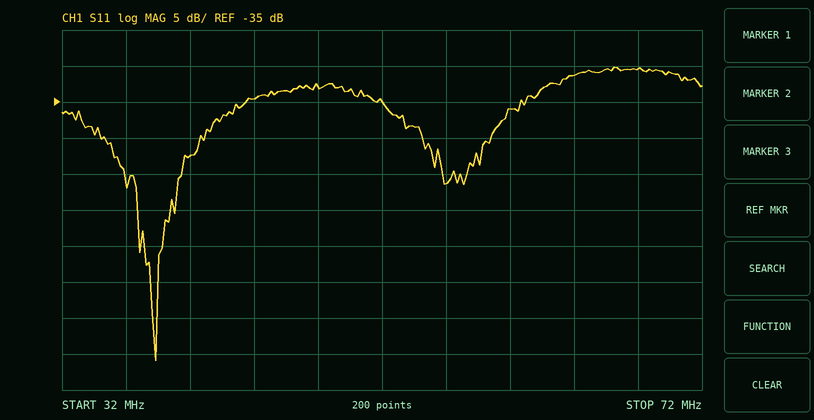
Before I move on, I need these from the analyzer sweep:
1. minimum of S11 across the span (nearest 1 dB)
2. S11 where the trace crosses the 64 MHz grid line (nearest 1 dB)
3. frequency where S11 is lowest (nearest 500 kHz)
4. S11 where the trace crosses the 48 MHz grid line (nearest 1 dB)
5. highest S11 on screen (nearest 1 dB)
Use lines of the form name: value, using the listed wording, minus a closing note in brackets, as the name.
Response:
minimum of S11 across the span: -71 dB
S11 where the trace crosses the 64 MHz grid line: -31 dB
frequency where S11 is lowest: 38.0 MHz
S11 where the trace crosses the 48 MHz grid line: -33 dB
highest S11 on screen: -30 dB
